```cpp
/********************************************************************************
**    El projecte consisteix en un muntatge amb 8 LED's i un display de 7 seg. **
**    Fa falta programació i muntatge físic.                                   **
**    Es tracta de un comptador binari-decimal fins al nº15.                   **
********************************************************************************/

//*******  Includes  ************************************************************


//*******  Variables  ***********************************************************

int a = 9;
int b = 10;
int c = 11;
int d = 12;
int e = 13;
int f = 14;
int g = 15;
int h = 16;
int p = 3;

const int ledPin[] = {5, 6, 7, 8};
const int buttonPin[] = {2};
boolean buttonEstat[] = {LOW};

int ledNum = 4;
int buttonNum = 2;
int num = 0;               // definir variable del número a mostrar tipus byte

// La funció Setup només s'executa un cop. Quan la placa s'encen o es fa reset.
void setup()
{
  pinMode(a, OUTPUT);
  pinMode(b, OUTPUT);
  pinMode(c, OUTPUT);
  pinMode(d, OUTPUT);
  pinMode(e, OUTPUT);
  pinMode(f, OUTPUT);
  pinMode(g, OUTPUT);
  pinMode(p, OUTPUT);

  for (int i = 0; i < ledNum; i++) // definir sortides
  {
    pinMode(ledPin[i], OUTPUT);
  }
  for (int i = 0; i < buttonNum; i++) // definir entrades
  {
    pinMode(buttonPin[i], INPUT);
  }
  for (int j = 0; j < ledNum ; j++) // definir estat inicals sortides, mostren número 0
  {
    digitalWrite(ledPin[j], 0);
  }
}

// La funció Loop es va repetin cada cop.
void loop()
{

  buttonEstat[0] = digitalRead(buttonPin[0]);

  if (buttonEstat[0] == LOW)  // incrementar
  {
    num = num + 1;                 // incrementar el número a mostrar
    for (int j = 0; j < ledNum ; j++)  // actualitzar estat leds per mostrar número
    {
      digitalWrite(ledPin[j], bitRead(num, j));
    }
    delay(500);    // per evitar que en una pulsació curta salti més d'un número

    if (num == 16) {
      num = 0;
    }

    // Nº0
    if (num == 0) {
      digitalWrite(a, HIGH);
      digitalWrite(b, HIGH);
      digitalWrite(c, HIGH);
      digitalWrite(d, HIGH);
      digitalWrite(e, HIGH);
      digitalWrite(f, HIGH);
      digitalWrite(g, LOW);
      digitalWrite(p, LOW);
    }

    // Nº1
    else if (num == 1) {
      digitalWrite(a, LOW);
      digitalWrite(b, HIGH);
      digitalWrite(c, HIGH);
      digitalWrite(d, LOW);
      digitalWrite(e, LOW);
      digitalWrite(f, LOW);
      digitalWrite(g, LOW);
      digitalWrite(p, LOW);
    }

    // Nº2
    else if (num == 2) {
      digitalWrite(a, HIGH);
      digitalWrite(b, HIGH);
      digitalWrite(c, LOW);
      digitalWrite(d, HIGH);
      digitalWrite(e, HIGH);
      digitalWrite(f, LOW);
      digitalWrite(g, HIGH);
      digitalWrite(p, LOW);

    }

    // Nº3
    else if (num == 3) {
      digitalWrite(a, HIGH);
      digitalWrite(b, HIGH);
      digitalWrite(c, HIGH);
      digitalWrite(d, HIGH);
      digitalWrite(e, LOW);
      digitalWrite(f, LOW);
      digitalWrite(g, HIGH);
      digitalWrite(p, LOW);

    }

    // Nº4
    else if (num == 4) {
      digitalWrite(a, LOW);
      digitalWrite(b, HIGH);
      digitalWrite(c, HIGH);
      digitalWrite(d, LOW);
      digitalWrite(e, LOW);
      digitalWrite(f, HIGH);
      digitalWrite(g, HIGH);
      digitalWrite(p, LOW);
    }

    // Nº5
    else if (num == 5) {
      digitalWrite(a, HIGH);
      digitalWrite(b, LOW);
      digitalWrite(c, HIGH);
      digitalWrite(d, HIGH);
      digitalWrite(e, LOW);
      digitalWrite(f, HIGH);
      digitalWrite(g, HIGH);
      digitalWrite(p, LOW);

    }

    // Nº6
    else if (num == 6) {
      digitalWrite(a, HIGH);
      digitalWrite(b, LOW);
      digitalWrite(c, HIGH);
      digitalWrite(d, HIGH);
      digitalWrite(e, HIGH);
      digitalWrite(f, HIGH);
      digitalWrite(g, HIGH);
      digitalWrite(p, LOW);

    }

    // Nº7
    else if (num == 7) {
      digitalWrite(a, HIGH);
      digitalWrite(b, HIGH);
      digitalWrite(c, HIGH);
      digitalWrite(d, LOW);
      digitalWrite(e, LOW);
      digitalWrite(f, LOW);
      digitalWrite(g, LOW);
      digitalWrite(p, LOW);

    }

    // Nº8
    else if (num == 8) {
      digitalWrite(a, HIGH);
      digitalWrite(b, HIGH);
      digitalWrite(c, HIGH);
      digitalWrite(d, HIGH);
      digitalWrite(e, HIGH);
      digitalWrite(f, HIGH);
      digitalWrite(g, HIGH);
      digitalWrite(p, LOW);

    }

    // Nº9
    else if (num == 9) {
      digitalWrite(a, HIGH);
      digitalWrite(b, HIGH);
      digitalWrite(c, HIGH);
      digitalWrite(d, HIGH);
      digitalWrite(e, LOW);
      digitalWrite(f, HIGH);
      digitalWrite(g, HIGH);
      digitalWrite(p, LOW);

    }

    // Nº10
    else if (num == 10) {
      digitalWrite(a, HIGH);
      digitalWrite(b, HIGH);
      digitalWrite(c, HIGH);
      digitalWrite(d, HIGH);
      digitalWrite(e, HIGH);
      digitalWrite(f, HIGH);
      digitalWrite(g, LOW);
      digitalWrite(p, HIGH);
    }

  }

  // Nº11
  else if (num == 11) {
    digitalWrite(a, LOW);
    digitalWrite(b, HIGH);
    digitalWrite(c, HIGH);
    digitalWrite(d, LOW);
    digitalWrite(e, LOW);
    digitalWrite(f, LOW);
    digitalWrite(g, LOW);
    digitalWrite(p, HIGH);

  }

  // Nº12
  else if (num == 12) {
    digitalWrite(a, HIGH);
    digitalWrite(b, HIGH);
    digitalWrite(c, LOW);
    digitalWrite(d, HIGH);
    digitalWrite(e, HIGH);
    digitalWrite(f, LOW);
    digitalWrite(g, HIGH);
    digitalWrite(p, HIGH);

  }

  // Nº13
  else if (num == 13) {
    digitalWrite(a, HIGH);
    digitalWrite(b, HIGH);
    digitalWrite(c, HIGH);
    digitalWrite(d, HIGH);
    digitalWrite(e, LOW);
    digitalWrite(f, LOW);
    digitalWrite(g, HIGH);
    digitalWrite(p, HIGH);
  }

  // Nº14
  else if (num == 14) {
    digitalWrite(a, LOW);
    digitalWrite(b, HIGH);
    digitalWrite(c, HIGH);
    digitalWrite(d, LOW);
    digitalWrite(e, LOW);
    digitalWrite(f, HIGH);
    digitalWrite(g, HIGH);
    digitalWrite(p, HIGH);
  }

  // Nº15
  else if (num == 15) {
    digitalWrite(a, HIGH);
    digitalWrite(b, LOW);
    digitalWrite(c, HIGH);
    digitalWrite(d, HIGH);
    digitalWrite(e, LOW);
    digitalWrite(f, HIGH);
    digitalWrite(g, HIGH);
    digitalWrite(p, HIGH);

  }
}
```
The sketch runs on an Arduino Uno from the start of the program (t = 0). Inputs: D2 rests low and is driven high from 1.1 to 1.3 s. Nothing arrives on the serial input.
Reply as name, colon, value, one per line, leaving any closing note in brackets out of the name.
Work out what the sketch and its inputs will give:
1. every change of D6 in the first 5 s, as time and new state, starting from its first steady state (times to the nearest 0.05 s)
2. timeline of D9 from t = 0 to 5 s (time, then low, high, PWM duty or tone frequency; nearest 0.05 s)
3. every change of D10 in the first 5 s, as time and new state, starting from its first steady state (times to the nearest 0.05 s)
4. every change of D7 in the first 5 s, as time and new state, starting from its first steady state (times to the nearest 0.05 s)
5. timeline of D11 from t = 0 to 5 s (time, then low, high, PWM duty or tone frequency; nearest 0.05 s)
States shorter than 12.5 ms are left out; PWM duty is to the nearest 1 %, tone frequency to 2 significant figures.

every change of D6 in the first 5 s, as time and new state, starting from its first steady state: 0 s low; 0.5 s high; 1.5 s low; 2.5 s high; 3.5 s low; 4.5 s high
timeline of D9 from t = 0 to 5 s: 0 s low; 1 s high; 2 s low; 2.5 s high
every change of D10 in the first 5 s, as time and new state, starting from its first steady state: 0 s low; 0.5 s high; 2.5 s low; 3.5 s high
every change of D7 in the first 5 s, as time and new state, starting from its first steady state: 0 s low; 1.5 s high; 3.5 s low
timeline of D11 from t = 0 to 5 s: 0 s low; 0.5 s high; 1 s low; 1.5 s high
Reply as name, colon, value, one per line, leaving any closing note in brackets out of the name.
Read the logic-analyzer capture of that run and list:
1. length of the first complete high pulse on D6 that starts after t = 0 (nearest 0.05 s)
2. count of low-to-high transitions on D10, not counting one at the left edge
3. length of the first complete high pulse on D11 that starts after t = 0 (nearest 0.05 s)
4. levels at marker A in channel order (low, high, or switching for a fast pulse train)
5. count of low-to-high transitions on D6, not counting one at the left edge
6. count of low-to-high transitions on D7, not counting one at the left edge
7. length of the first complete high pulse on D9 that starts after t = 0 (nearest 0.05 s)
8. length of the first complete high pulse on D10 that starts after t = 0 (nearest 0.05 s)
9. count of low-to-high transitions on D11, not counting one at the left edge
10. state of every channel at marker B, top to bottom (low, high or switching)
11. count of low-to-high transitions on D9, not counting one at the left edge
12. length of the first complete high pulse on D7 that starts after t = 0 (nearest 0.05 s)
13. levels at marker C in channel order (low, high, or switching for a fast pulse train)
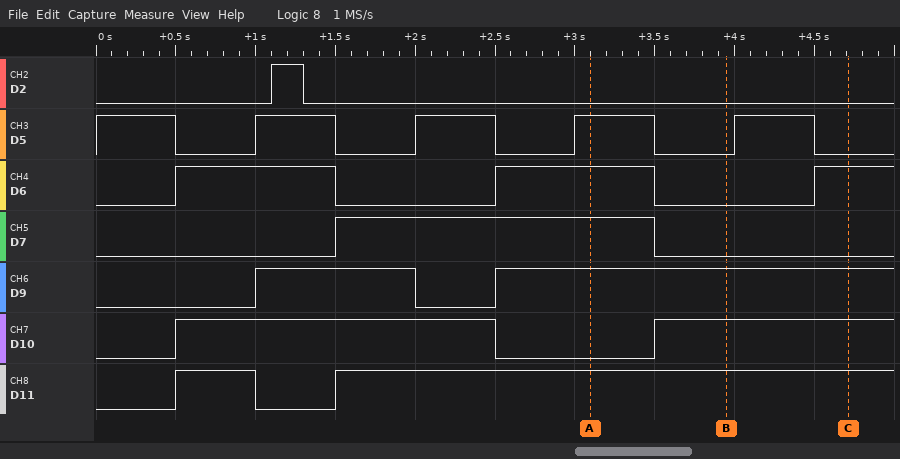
length of the first complete high pulse on D6 that starts after t = 0: 1.00 s
count of low-to-high transitions on D10, not counting one at the left edge: 2
length of the first complete high pulse on D11 that starts after t = 0: 0.50 s
levels at marker A in channel order: D2 low, D5 high, D6 high, D7 high, D9 high, D10 low, D11 high
count of low-to-high transitions on D6, not counting one at the left edge: 3
count of low-to-high transitions on D7, not counting one at the left edge: 1
length of the first complete high pulse on D9 that starts after t = 0: 1.00 s
length of the first complete high pulse on D10 that starts after t = 0: 2.00 s
count of low-to-high transitions on D11, not counting one at the left edge: 2
state of every channel at marker B, top to bottom: D2 low, D5 low, D6 low, D7 low, D9 high, D10 high, D11 high
count of low-to-high transitions on D9, not counting one at the left edge: 2
length of the first complete high pulse on D7 that starts after t = 0: 2.00 s
levels at marker C in channel order: D2 low, D5 low, D6 high, D7 low, D9 high, D10 high, D11 high
